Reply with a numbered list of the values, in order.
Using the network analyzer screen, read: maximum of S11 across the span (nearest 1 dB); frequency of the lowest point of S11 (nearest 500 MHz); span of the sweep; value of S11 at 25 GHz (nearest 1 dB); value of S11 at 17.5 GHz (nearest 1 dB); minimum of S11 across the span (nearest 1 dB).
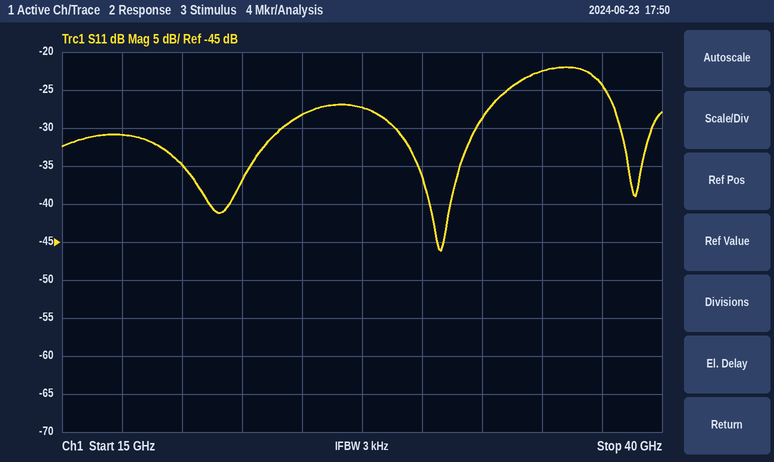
1. -22 dB
2. 31.0 GHz
3. 25 GHz
4. -28 dB
5. -31 dB
6. -46 dB
